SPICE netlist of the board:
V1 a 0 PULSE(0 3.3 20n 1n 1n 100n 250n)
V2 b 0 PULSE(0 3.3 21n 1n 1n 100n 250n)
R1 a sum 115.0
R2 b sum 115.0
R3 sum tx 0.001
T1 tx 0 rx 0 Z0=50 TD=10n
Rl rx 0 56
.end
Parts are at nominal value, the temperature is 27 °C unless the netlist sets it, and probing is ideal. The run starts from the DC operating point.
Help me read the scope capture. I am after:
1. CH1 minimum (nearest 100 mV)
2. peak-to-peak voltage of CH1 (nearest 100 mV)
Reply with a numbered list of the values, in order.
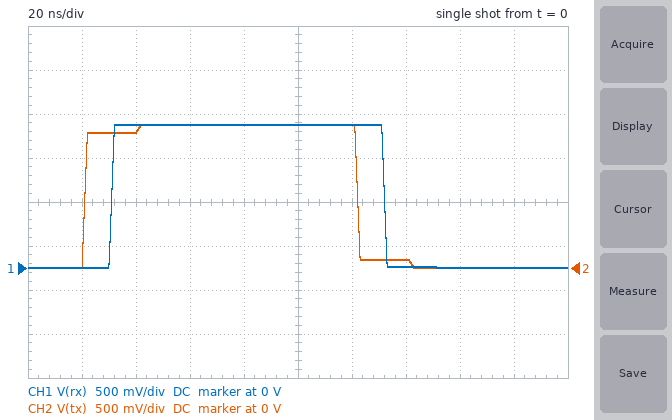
1. 0 V
2. 1.6 V
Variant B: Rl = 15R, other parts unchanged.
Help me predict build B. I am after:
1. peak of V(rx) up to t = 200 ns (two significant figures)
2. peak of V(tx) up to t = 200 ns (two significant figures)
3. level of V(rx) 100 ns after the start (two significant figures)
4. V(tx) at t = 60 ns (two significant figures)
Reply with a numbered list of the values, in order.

1. 710 mV
2. 1.5 V
3. 680 mV
4. 650 mV
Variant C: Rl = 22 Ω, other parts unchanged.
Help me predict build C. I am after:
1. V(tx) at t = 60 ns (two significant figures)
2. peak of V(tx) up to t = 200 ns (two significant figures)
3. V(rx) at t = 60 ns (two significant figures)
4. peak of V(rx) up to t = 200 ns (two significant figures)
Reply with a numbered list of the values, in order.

1. 900 mV
2. 1.5 V
3. 910 mV
4. 940 mV
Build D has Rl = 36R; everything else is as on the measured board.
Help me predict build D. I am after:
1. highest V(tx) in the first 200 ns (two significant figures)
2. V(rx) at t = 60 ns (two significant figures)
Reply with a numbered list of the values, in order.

1. 1.5 V
2. 1.3 V
